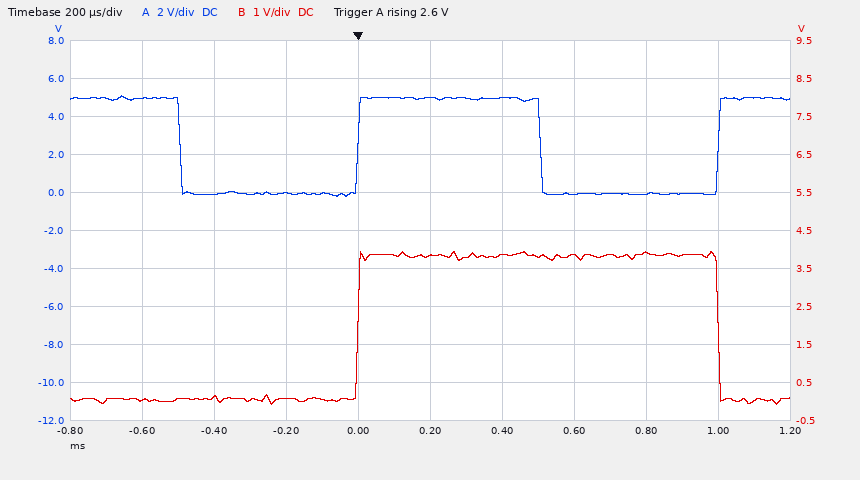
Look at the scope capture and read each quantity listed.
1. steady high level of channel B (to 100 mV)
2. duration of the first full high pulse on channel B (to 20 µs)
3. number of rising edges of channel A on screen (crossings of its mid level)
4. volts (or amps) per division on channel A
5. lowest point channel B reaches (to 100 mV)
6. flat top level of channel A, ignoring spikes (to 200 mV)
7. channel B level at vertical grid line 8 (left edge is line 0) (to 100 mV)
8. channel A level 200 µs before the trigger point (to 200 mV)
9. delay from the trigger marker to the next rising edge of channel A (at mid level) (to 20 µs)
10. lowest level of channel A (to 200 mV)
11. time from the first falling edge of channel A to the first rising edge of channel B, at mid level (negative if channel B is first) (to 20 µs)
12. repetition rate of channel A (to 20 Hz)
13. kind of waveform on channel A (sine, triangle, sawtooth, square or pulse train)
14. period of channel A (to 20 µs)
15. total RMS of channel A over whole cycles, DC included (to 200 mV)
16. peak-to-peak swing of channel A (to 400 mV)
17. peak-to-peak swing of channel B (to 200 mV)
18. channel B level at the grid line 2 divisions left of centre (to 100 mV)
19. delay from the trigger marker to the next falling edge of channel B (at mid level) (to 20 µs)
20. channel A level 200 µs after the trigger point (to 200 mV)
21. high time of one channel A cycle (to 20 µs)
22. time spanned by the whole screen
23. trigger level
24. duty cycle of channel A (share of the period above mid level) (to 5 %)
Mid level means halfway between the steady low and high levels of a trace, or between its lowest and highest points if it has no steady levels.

3.9 V
1.00 ms
2
2 V
-100 mV
5.0 V
3.9 V
0.0 V
1.00 ms
-200 mV
+500 µs
1.00 kHz
square
1.00 ms
3.6 V
5.2 V
4.0 V
100 mV
1.00 ms
5.0 V
500 µs
2 ms
2.6 V
50 %
